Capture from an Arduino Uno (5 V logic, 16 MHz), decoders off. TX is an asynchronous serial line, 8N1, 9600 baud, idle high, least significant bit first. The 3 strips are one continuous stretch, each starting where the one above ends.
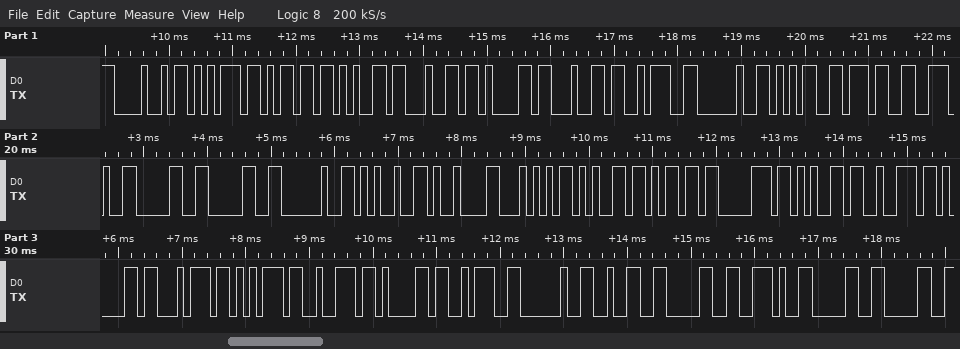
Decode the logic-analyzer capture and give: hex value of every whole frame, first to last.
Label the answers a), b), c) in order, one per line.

a) 48 75 6D 65 64 61 64 3A 20 35 37 2E 30 30 20 25 09 54 65 6D 70 65 72 61 74 75 72 61 3A 20 32 30 2E 30 30
